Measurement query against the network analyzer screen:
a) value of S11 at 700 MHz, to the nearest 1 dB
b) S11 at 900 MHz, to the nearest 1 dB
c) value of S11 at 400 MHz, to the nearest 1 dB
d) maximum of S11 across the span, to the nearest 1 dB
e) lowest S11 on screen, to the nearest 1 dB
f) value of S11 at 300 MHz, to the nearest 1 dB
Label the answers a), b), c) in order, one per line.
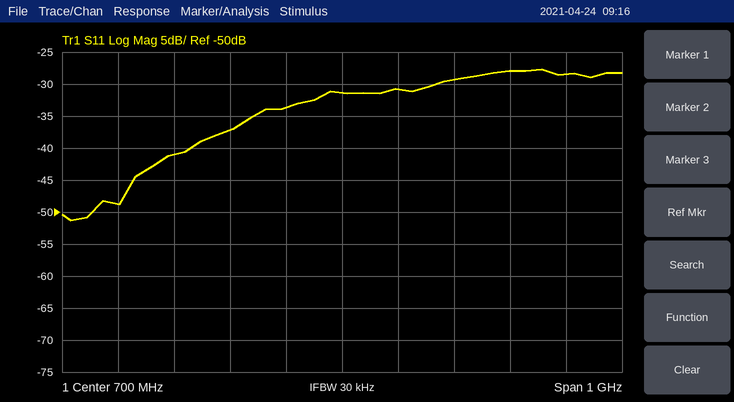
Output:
a) -31 dB
b) -29 dB
c) -41 dB
d) -28 dB
e) -51 dB
f) -49 dB
